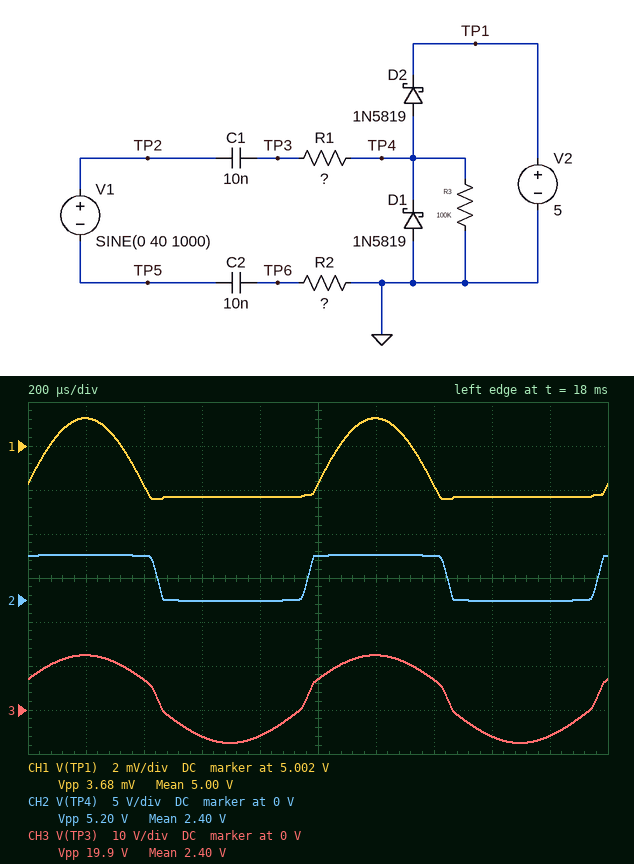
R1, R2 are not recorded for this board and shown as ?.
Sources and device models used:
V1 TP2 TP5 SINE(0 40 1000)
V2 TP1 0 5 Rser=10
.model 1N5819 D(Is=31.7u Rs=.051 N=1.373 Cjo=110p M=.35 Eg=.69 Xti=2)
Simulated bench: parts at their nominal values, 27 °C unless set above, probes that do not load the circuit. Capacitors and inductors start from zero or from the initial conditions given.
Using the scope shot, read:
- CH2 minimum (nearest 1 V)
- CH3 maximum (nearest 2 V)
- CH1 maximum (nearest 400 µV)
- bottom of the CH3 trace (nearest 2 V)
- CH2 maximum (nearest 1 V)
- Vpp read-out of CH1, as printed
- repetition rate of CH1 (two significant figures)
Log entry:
0 V
12 V
5.0032 V
-8 V
5 V
3.68 mV
1.0 kHz
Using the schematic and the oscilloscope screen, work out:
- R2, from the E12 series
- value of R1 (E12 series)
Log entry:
68 kΩ
18 kΩ
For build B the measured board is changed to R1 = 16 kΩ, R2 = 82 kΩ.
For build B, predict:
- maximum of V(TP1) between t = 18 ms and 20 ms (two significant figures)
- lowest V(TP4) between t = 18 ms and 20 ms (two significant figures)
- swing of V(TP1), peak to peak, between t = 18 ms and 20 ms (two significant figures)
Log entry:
5.0 V
-87 mV
3.2 mV
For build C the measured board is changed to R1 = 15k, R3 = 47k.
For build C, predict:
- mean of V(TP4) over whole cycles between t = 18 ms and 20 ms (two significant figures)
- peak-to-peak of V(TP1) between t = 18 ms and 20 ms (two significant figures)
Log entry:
2.3 V
3.2 mV
